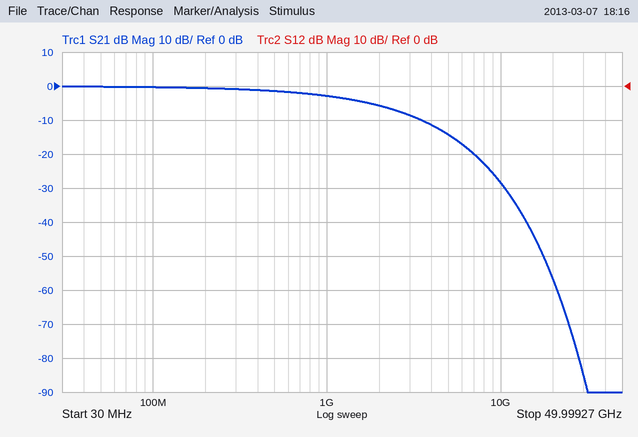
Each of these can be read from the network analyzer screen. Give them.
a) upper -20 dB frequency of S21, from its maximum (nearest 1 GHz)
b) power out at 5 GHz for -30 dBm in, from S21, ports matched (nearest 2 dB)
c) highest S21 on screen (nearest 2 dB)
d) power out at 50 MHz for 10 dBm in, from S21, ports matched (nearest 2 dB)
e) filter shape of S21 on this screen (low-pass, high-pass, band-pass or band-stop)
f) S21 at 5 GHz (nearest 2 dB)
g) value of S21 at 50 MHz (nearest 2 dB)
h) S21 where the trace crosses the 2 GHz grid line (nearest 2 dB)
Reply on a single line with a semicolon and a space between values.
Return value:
7 GHz; -44 dBm; 0 dB; 10 dBm; low-pass; -14 dB; 0 dB; -6 dB
